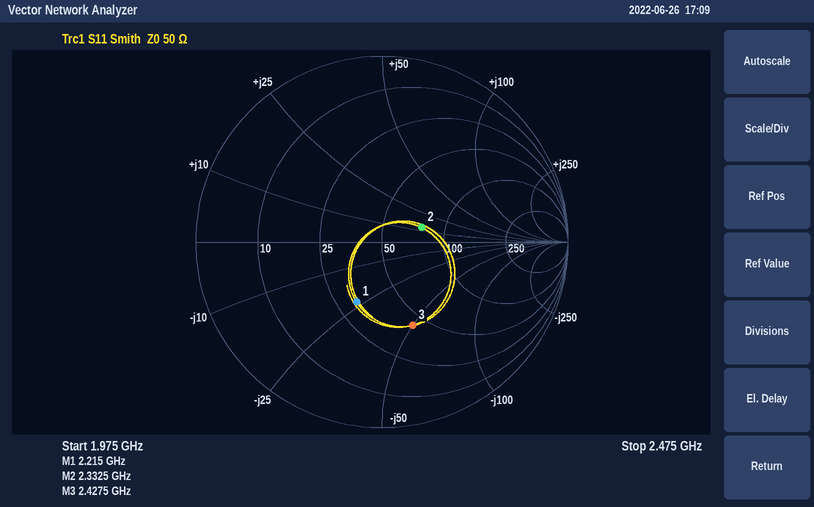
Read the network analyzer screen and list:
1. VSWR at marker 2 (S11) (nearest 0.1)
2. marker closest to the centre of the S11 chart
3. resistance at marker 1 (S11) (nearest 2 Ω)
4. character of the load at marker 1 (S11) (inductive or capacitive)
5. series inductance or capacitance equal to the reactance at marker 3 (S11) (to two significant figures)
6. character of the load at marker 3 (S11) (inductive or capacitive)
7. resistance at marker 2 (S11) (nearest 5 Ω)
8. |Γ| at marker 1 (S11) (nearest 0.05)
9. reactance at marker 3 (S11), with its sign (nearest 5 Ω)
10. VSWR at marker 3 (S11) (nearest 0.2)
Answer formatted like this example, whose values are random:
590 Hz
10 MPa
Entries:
1.6
marker 2
32 Ω
capacitive
1.3 pF
capacitive
75 Ω
0.35
-50 Ω
2.8
